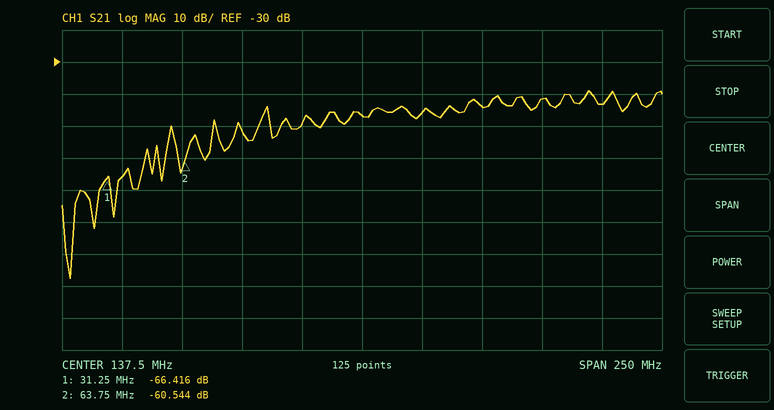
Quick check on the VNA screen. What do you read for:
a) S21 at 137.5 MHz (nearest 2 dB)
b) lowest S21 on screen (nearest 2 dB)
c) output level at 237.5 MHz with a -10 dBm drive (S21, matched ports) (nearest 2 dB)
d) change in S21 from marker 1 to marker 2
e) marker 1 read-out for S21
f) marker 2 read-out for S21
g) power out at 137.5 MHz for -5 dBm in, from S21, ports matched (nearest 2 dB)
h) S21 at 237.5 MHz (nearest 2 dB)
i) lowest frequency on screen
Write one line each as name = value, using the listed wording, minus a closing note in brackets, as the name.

S21 at 137.5 MHz = -46 dB
lowest S21 on screen = -98 dB
output level at 237.5 MHz with a -10 dBm drive (S21, matched ports) = -54 dBm
change in S21 from marker 1 to marker 2 = 5.872 dB
marker 1 read-out for S21 = -66.416 dB
marker 2 read-out for S21 = -60.544 dB
power out at 137.5 MHz for -5 dBm in, from S21, ports matched = -52 dBm
S21 at 237.5 MHz = -44 dB
lowest frequency on screen = 12.5 MHz
